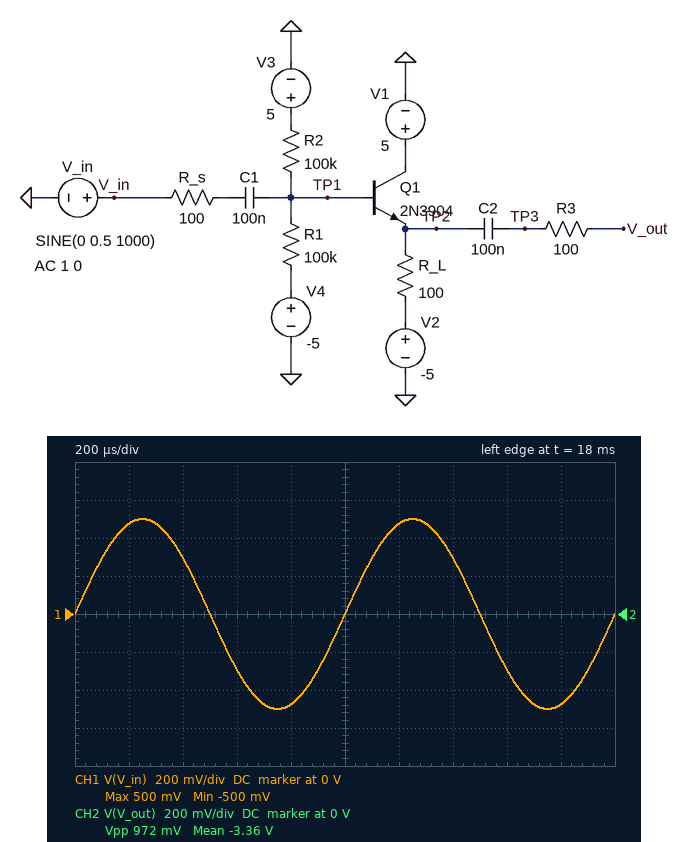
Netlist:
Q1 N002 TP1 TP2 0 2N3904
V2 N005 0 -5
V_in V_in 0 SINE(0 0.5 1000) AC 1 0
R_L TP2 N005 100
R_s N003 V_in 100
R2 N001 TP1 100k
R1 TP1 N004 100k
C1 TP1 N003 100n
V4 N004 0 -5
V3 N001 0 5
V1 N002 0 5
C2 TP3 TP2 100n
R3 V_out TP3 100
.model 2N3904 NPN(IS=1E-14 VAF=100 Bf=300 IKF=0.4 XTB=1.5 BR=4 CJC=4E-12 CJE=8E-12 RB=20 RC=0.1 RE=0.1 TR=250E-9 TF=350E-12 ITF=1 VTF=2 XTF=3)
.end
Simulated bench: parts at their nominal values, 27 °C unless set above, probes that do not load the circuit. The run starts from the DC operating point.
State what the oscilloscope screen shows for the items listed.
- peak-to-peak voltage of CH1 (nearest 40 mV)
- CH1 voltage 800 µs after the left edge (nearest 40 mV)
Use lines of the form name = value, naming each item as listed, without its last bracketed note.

peak-to-peak voltage of CH1 = 1.00 V
CH1 voltage 800 µs after the left edge = -480 mV
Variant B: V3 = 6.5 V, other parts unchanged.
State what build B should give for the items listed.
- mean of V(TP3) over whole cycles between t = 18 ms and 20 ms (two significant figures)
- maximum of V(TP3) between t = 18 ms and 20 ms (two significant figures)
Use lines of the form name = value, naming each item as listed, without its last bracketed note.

mean of V(TP3) over whole cycles between t = 18 ms and 20 ms = -3.1 V
maximum of V(TP3) between t = 18 ms and 20 ms = -2.6 V
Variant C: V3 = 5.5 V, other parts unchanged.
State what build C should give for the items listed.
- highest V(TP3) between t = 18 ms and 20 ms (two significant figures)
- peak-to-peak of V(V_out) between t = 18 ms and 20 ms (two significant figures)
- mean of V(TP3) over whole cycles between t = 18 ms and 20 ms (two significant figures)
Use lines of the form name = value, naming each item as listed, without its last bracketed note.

highest V(TP3) between t = 18 ms and 20 ms = -2.8 V
peak-to-peak of V(V_out) between t = 18 ms and 20 ms = 970 mV
mean of V(TP3) over whole cycles between t = 18 ms and 20 ms = -3.3 V
